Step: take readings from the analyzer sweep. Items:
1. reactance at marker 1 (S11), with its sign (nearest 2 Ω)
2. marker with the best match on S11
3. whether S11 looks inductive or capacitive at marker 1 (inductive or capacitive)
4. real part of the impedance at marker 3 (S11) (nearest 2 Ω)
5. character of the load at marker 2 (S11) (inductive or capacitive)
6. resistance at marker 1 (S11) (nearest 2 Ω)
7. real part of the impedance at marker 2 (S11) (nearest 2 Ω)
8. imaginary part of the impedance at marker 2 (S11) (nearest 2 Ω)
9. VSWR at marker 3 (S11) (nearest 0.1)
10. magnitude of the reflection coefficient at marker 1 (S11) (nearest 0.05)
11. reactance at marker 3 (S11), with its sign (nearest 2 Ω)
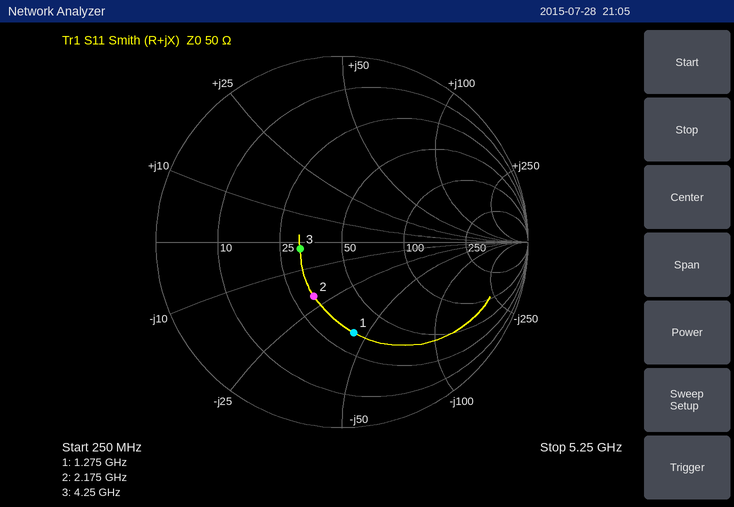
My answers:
-44 Ω
marker 3
capacitive
32 Ω
capacitive
34 Ω
32 Ω
-20 Ω
1.6
0.50
-2 Ω
